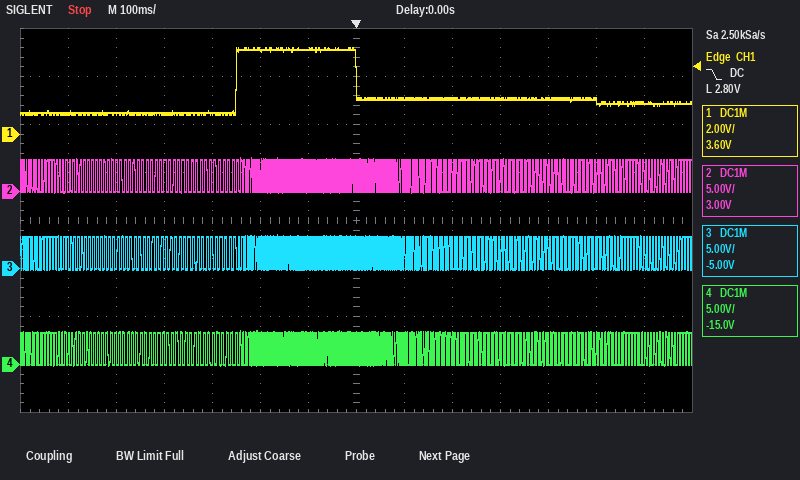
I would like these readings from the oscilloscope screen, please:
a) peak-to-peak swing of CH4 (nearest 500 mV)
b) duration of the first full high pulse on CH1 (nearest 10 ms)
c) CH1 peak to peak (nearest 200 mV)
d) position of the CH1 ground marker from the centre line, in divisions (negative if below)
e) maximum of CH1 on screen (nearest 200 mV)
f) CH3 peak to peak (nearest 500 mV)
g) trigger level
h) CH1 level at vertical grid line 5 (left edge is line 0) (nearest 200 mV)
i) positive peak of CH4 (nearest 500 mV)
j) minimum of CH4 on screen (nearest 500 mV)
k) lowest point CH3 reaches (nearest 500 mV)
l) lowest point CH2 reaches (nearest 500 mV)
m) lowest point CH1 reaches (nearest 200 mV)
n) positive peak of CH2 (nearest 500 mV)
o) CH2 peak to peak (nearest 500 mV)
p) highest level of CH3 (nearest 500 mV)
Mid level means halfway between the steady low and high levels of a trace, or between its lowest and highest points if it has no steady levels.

3.5 V
250 ms
2.8 V
+1.8 div
3.6 V
3.5 V
2.80 V
3.6 V
3.5 V
0.0 V
0.0 V
0.0 V
800 mV
3.5 V
3.5 V
3.5 V
